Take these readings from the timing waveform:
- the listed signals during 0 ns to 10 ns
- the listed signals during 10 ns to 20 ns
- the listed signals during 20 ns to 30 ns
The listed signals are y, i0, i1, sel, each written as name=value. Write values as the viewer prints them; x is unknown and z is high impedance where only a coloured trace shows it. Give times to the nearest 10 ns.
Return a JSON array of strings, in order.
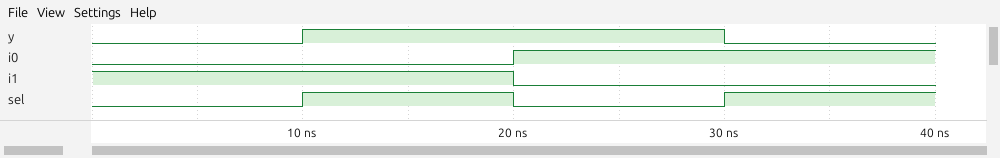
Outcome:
["y=0, i0=0, i1=1, sel=0", "y=1, i0=0, i1=1, sel=1", "y=1, i0=1, i1=0, sel=0"]
